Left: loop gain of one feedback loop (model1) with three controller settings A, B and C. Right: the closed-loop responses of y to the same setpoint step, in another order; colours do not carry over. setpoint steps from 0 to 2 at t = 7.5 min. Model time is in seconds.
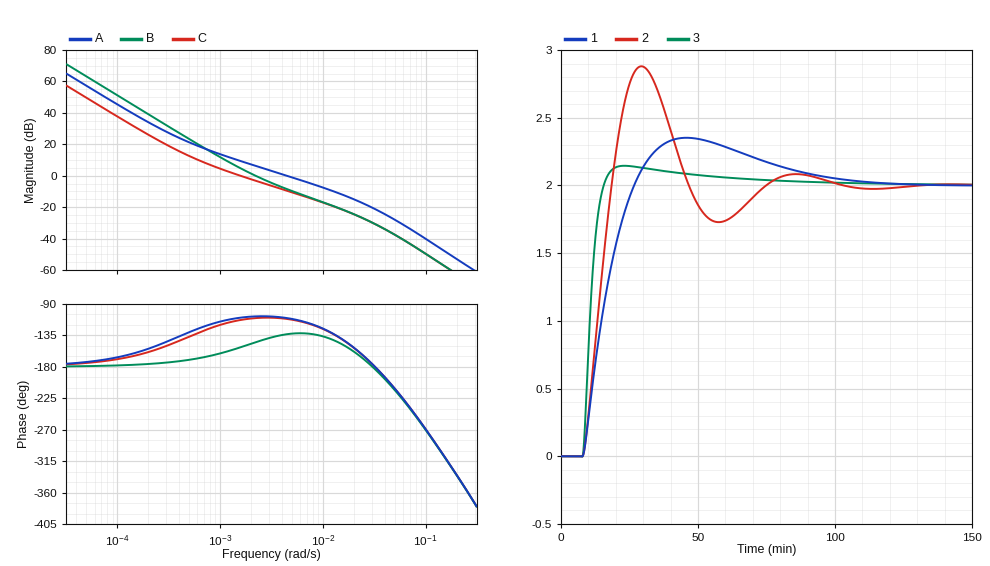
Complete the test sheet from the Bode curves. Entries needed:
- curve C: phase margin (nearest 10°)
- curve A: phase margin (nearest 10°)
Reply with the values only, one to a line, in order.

70°
70°
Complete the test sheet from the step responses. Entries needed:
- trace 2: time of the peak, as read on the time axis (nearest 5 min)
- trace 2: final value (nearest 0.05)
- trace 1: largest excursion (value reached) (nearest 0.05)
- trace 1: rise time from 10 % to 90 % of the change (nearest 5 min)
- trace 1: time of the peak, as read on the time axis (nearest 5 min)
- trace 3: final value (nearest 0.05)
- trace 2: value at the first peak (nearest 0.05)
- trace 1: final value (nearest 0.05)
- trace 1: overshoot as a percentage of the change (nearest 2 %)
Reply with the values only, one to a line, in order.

30 min
2.00
2.35
15 min
45 min
2.00
2.90
2.00
18 %
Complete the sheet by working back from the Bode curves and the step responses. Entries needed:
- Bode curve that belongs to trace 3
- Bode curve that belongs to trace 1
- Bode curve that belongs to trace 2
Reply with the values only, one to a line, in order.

A
C
B
